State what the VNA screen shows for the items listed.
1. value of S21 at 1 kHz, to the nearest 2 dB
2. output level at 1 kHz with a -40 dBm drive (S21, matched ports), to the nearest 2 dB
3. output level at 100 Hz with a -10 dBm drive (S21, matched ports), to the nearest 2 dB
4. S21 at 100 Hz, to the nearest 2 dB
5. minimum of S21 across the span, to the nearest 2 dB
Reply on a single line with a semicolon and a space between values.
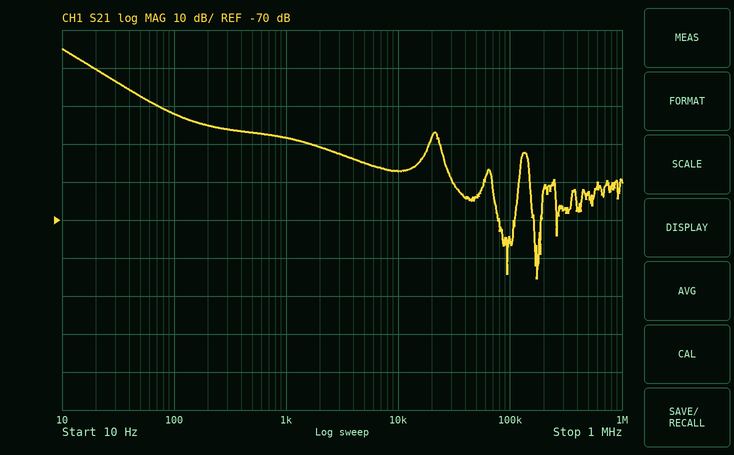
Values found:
-48 dB; -88 dBm; -52 dBm; -42 dB; -86 dB
